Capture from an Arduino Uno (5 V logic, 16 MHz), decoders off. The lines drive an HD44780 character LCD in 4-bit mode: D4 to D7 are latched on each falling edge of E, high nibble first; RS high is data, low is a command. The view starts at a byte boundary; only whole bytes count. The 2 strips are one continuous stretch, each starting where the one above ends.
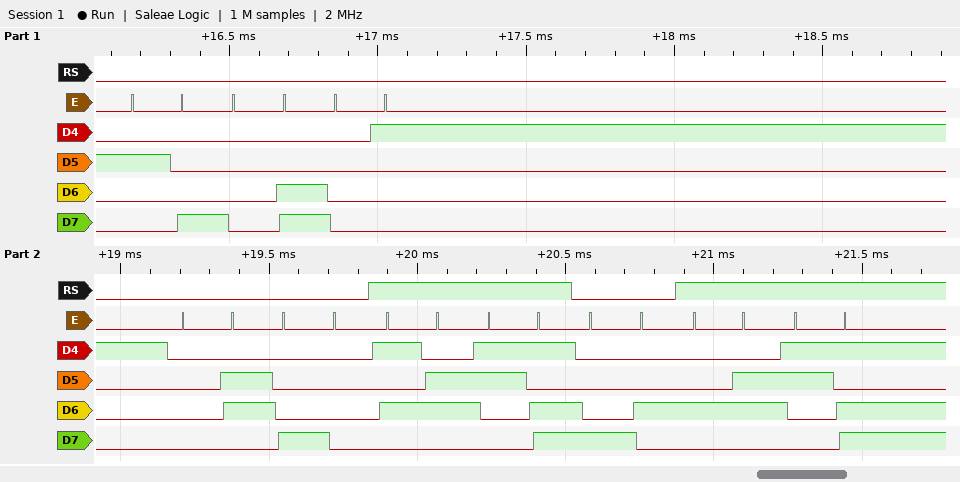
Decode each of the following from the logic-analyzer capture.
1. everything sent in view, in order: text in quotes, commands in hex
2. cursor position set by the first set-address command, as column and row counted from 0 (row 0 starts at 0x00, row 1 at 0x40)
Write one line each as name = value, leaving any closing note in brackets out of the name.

everything sent in view, in order: text in quotes, commands in hex = 0x28 0x0C 0x01 0x06 0x80 "V=" 0x84 "F="
cursor position set by the first set-address command, as column and row counted from 0 = column 0, row 0
